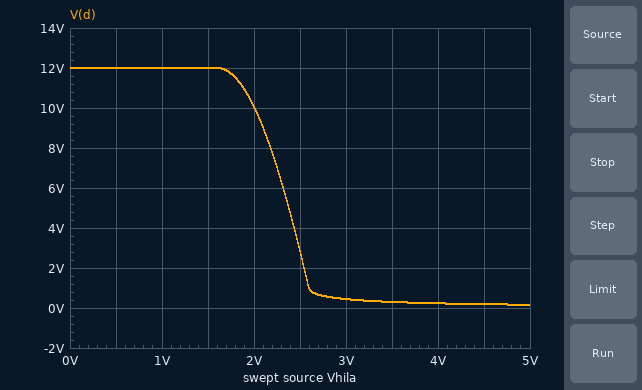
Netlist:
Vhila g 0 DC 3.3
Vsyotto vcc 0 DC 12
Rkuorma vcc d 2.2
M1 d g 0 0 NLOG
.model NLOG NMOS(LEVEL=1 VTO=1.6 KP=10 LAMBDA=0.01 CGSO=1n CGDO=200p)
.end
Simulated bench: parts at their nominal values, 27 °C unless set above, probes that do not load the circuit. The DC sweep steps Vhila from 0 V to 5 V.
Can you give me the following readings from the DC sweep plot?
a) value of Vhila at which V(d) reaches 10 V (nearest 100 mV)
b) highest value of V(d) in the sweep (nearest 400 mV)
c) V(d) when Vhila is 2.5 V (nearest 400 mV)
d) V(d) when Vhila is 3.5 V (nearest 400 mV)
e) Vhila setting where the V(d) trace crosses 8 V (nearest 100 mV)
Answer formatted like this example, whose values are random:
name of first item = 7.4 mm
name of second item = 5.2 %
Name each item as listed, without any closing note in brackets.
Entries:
value of Vhila at which V(d) reaches 10 V = 2.0 V
highest value of V(d) in the sweep = 12.0 V
V(d) when Vhila is 2.5 V = 2.8 V
V(d) when Vhila is 3.5 V = 400 mV
Vhila setting where the V(d) trace crosses 8 V = 2.2 V
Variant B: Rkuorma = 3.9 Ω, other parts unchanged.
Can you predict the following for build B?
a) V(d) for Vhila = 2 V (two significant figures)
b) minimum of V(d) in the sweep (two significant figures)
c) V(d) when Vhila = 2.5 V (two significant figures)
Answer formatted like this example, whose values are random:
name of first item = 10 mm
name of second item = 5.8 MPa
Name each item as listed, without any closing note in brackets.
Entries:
V(d) for Vhila = 2 V = 8.6 V
minimum of V(d) in the sweep = 91 mV
V(d) when Vhila = 2.5 V = 430 mV
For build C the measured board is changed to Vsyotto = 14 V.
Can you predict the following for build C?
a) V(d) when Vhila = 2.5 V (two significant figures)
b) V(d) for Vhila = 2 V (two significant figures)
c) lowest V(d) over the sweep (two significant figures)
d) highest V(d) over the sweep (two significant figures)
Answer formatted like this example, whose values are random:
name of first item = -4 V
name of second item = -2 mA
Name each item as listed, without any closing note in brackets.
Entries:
V(d) when Vhila = 2.5 V = 4.7 V
V(d) for Vhila = 2 V = 12 V
lowest V(d) over the sweep = 190 mV
highest V(d) over the sweep = 14 V
